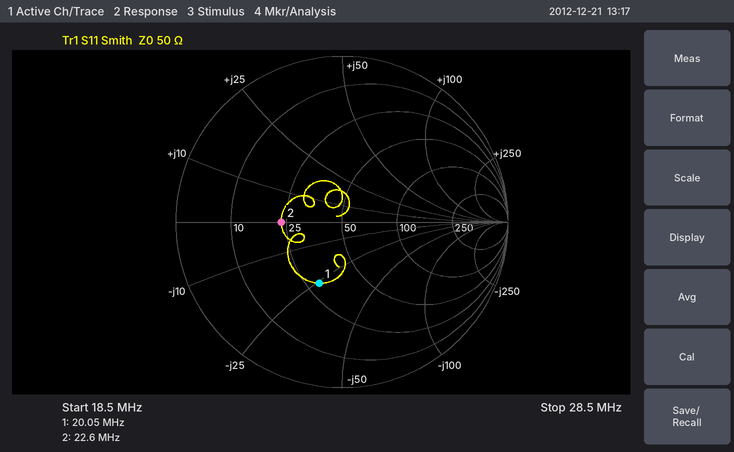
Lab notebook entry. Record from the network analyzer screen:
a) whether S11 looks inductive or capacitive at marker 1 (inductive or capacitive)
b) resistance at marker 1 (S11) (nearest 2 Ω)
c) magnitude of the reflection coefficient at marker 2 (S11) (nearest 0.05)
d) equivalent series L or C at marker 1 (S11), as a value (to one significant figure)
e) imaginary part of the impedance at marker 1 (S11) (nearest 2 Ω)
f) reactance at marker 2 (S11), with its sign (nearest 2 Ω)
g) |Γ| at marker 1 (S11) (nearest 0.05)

capacitive
30 Ω
0.35
300 pF
-26 Ω
0 Ω
0.40
